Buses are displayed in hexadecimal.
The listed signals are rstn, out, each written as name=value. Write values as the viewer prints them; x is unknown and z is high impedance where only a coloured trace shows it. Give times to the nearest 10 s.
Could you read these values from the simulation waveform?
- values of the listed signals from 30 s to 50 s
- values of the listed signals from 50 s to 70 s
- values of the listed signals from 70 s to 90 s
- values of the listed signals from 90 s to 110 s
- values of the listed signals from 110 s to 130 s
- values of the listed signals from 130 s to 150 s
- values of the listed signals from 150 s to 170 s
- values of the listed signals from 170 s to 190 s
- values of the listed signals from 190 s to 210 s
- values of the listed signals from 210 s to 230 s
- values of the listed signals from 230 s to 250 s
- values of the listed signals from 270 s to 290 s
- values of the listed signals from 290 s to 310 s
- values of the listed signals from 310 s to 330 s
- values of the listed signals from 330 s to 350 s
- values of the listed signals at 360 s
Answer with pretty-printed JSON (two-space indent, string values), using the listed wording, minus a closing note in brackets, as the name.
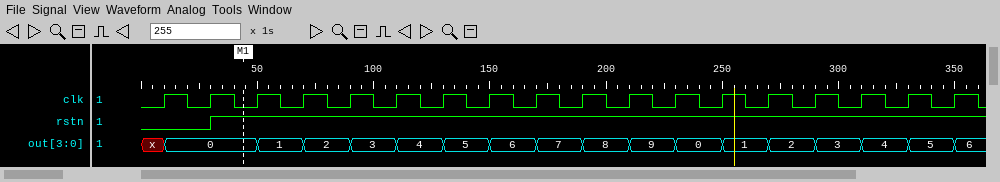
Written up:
{
  "values of the listed signals from 30 s to 50 s": "rstn=1, out=0",
  "values of the listed signals from 50 s to 70 s": "rstn=1, out=1",
  "values of the listed signals from 70 s to 90 s": "rstn=1, out=2",
  "values of the listed signals from 90 s to 110 s": "rstn=1, out=3",
  "values of the listed signals from 110 s to 130 s": "rstn=1, out=4",
  "values of the listed signals from 130 s to 150 s": "rstn=1, out=5",
  "values of the listed signals from 150 s to 170 s": "rstn=1, out=6",
  "values of the listed signals from 170 s to 190 s": "rstn=1, out=7",
  "values of the listed signals from 190 s to 210 s": "rstn=1, out=8",
  "values of the listed signals from 210 s to 230 s": "rstn=1, out=9",
  "values of the listed signals from 230 s to 250 s": "rstn=1, out=0",
  "values of the listed signals from 270 s to 290 s": "rstn=1, out=2",
  "values of the listed signals from 290 s to 310 s": "rstn=1, out=3",
  "values of the listed signals from 310 s to 330 s": "rstn=1, out=4",
  "values of the listed signals from 330 s to 350 s": "rstn=1, out=5",
  "values of the listed signals at 360 s": "rstn=1, out=6"
}
